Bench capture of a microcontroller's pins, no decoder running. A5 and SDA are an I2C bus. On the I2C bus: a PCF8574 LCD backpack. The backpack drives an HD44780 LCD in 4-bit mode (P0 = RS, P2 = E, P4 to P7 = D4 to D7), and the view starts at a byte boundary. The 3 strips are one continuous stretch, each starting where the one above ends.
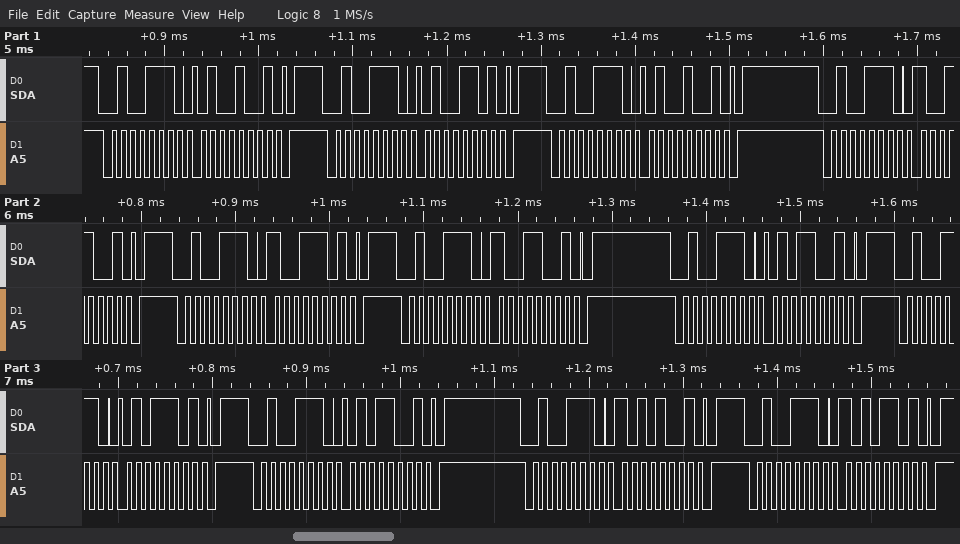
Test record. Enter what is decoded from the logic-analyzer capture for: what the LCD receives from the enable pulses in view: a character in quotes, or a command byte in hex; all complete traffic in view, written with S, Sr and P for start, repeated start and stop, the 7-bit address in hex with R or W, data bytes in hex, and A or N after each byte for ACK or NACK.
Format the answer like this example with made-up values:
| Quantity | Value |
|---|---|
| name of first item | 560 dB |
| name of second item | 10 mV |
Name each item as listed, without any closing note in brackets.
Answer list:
| Quantity | Value |
|---|---|
| what the LCD receives from the enable pulses in view: a character in quotes, or a command byte in hex | 'I' |
| all complete traffic in view, written with S, Sr and P for start, repeated start and stop, the 7-bit address in hex with R or W, data bytes in hex, and A or N after each byte for ACK or NACK | S 27W A 49 A P S 27W A 4D A P S 27W A 49 A P S 27W A 99 A P S 27W A 9D A P S 27W A 99 A P S 27W A 59 A P S 27W A 5D A P S 27W A 59 A P S 27W A A9 A P S 27W A AD A P |
